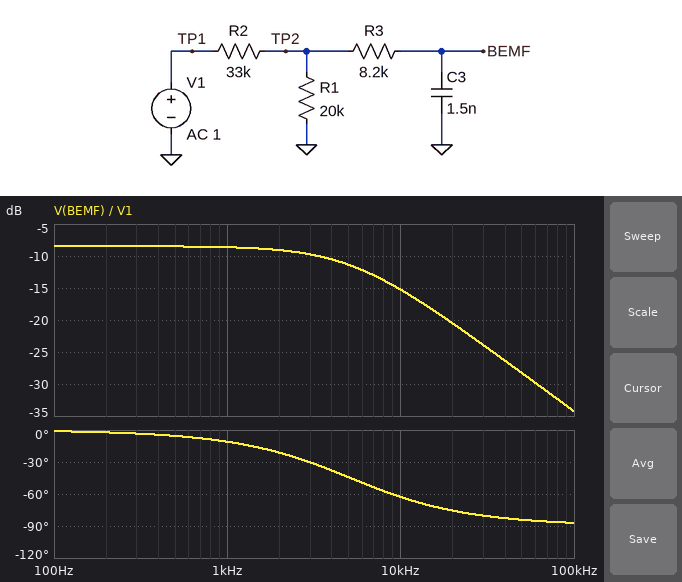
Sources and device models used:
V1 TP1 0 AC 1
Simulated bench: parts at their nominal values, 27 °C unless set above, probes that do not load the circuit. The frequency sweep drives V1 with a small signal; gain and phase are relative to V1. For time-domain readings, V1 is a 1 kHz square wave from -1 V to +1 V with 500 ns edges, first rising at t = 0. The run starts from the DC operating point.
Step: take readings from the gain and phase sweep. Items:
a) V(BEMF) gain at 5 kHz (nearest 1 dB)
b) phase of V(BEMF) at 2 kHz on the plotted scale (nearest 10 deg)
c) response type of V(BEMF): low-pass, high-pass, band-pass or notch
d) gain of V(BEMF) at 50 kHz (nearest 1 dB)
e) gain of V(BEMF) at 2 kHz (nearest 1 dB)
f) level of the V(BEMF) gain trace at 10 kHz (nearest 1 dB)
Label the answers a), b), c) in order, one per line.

a) -11 dB
b) -20 deg
c) low-pass
d) -28 dB
e) -9 dB
f) -15 dB
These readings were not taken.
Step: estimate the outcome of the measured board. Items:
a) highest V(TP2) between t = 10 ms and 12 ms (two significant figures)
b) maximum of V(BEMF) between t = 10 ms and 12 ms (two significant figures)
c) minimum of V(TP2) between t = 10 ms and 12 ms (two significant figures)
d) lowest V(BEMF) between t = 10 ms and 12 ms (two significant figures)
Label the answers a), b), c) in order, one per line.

a) 380 mV
b) 380 mV
c) -380 mV
d) -380 mV
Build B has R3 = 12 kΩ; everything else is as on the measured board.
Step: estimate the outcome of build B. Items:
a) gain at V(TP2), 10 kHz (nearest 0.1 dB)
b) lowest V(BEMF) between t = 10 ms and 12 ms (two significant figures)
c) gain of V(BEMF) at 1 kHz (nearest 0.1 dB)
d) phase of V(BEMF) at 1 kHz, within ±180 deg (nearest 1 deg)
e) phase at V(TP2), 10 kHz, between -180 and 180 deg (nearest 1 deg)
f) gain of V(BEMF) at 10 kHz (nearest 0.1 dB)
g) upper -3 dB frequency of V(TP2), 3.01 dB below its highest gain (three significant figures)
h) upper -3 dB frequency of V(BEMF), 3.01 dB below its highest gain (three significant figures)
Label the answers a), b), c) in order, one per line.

a) -12.9 dB
b) -380 mV
c) -8.7 dB
d) -13 deg
e) -18 deg
f) -16.5 dB
g) 6.03 kHz
h) 4.34 kHz
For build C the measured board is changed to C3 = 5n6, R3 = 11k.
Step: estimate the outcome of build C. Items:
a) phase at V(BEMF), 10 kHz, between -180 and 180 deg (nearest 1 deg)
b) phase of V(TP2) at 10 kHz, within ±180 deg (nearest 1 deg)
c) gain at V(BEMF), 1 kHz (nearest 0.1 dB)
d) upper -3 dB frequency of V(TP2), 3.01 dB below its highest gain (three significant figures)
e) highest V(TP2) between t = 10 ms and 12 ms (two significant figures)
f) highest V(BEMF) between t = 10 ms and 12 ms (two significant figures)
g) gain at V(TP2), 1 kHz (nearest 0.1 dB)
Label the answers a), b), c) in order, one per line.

a) -83 deg
b) -8 deg
c) -10.7 dB
d) 1.62 kHz
e) 370 mV
f) 360 mV
g) -10.1 dB
